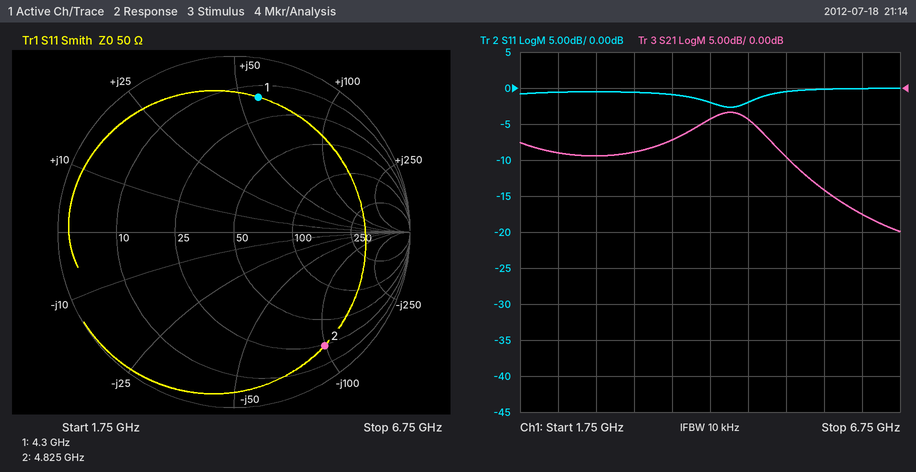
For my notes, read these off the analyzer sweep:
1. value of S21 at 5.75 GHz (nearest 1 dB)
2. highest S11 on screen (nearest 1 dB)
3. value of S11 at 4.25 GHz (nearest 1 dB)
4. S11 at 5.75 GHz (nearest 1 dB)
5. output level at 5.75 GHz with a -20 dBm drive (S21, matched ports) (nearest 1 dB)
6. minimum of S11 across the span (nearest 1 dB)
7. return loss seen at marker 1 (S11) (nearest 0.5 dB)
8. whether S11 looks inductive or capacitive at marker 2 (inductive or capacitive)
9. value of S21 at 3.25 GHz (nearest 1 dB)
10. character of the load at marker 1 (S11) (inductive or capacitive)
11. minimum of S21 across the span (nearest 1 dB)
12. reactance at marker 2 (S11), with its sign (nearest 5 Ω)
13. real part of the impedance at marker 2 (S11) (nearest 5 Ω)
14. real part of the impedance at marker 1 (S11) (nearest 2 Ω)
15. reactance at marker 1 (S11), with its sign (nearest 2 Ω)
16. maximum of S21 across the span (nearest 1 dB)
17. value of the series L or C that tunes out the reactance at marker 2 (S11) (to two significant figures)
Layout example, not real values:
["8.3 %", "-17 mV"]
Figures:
["-14 dB", "0 dB", "-2 dB", "0 dB", "-34 dBm", "-3 dB", "2.0 dB", "capacitive", "-9 dB", "inductive", "-20 dB", "-100 Ω", "25 Ω", "14 Ω", "+58 Ω", "-3 dB", "3.3 nH"]
